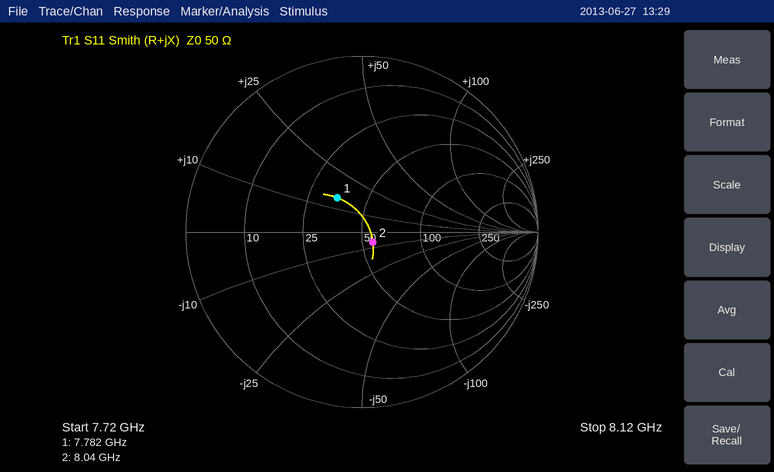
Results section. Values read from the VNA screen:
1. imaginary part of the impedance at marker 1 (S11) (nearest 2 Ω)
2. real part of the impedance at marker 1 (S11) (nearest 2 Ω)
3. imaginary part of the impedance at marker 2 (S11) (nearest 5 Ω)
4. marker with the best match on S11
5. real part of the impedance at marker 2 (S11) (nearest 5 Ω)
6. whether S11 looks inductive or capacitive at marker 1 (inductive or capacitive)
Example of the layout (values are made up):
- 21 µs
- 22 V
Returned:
- +14 Ω
- 36 Ω
- -5 Ω
- marker 2
- 55 Ω
- inductive
